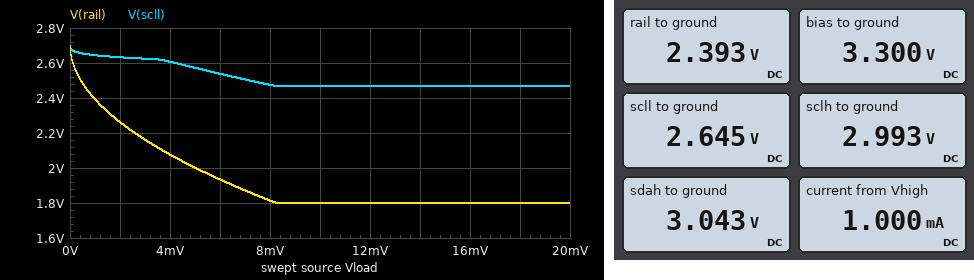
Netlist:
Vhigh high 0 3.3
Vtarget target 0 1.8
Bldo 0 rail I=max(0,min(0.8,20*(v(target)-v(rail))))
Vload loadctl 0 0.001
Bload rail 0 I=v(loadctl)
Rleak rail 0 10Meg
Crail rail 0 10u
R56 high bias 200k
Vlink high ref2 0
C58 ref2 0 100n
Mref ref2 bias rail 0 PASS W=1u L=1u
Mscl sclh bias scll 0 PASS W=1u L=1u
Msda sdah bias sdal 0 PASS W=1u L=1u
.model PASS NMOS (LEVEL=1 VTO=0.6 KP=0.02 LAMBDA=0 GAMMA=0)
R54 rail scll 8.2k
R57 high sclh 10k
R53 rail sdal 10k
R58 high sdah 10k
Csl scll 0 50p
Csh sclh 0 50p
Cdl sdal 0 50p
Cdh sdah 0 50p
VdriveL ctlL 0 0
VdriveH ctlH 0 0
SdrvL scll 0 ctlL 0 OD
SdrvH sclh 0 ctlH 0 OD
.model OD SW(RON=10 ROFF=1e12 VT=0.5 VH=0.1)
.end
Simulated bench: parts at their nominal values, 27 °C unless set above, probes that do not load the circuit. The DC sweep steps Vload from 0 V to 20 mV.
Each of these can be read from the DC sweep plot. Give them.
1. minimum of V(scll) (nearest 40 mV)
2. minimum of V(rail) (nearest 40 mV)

2.48 V
1.80 V
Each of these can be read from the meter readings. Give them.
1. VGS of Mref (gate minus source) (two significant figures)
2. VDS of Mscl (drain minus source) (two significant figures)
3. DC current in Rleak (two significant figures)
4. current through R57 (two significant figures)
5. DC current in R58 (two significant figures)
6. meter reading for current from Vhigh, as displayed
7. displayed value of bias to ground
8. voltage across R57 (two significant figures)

910 mV
350 mV
240 nA
31 µA
26 µA
1.000 mA
3.300 V
310 mV
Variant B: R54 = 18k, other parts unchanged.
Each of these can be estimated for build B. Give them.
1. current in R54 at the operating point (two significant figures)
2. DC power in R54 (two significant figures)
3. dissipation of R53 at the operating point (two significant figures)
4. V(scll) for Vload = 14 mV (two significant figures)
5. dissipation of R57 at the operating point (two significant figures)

15 µA
4.1 µW
6.7 µW
2.6 V
2.3 µW
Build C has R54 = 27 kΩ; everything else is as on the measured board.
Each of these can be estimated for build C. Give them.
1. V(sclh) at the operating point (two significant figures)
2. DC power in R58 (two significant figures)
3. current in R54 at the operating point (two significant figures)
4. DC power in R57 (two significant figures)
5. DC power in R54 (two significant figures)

3.2 V
6.7 µW
10 µA
1.1 µW
2.9 µW
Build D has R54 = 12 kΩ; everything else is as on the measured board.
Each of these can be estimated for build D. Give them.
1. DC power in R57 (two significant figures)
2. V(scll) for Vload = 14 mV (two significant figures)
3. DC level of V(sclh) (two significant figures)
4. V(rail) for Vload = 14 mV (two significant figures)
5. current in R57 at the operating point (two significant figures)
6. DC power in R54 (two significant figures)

4.8 µW
2.6 V
3.1 V
1.8 V
22 µA
5.7 µW
